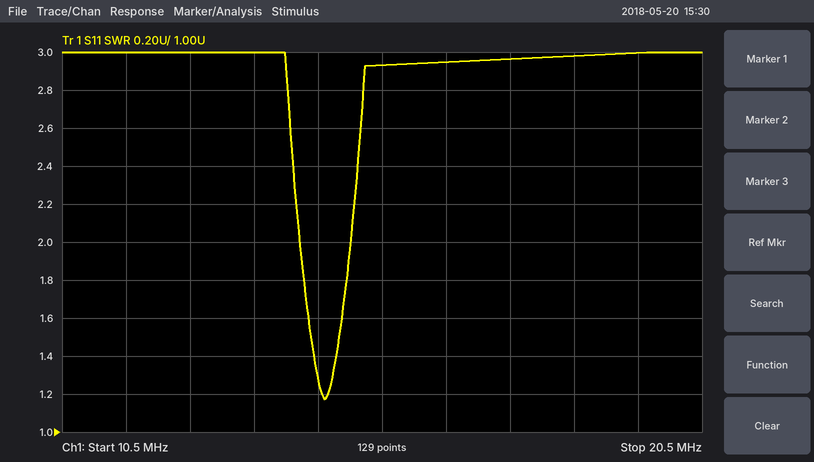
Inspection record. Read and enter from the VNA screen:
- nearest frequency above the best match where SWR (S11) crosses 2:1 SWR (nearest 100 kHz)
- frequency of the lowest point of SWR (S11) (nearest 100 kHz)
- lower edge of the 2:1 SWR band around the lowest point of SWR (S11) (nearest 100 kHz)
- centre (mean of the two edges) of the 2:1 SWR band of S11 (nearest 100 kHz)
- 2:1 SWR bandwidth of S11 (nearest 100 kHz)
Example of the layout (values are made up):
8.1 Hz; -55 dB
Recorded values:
15.0 MHz; 14.6 MHz; 14.2 MHz; 14.6 MHz; 800 kHz
